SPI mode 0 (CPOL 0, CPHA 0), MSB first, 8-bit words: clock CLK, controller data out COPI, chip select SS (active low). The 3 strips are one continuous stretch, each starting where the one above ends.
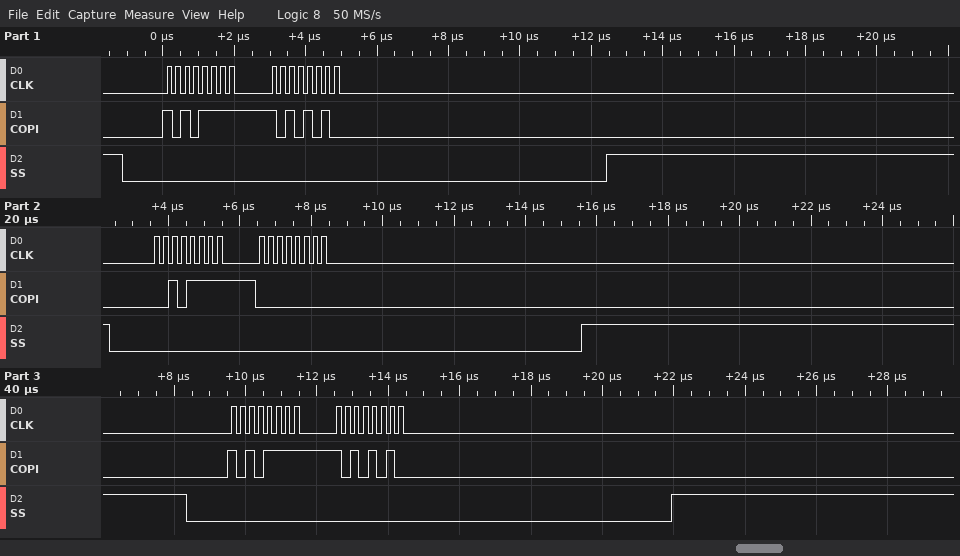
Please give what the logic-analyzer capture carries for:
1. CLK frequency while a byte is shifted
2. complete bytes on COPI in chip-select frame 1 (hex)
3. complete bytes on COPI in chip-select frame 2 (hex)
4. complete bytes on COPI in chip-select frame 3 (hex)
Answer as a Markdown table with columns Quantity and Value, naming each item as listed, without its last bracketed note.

| Quantity | Value |
|---|---|
| CLK frequency while a byte is shifted | 4 MHz |
| complete bytes on COPI in chip-select frame 1 | AF AA |
| complete bytes on COPI in chip-select frame 2 | 2F 00 |
| complete bytes on COPI in chip-select frame 3 | AF AA |
